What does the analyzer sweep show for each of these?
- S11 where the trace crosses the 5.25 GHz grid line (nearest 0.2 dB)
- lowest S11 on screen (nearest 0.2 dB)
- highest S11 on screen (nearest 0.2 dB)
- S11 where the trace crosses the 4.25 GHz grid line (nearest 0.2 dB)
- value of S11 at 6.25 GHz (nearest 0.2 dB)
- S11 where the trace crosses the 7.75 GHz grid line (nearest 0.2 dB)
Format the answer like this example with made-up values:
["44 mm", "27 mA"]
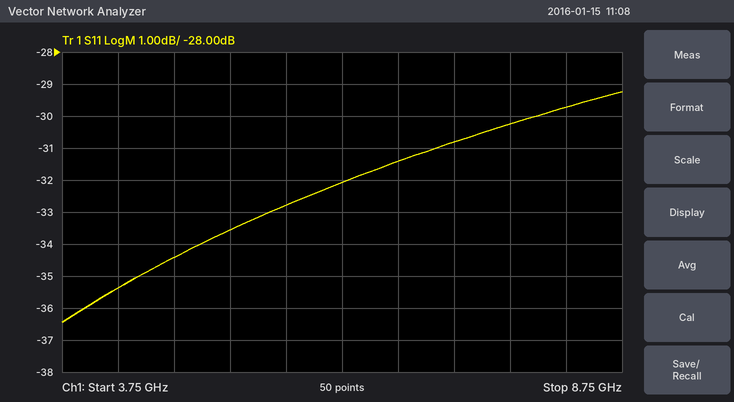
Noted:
["-33.6 dB", "-36.4 dB", "-29.2 dB", "-35.4 dB", "-32.0 dB", "-30.2 dB"]
